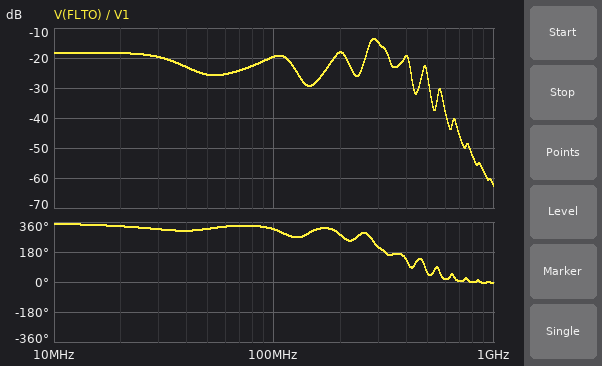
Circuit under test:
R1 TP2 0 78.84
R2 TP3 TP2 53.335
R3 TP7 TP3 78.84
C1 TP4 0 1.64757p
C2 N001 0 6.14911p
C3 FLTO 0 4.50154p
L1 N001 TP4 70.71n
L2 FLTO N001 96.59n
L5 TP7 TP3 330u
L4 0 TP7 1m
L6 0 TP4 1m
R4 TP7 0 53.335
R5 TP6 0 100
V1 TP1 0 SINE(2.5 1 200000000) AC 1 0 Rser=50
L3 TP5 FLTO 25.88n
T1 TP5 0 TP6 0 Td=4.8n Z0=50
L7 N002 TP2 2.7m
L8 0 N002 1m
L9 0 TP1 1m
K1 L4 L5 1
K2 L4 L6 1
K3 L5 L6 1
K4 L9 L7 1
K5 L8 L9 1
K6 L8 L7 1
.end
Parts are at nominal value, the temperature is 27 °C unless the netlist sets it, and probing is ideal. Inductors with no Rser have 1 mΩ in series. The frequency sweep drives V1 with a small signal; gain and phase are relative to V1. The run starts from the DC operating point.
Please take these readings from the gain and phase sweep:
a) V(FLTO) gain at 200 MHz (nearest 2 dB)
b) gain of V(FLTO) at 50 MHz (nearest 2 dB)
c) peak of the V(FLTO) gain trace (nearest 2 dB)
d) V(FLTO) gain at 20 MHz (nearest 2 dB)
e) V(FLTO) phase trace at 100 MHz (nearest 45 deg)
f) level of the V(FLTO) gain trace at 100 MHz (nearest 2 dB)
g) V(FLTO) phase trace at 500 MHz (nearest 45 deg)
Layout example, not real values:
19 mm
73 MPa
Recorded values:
-18 dB
-26 dB
-14 dB
-18 dB
315 deg
-20 dB
45 deg
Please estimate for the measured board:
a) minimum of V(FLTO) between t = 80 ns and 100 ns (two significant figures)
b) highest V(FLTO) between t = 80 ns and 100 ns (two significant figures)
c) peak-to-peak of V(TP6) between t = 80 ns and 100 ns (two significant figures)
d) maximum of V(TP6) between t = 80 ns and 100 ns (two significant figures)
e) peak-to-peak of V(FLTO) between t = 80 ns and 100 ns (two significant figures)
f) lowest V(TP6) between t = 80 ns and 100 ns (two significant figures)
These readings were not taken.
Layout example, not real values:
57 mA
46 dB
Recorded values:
-120 mV
120 mV
220 mV
110 mV
250 mV
-110 mV
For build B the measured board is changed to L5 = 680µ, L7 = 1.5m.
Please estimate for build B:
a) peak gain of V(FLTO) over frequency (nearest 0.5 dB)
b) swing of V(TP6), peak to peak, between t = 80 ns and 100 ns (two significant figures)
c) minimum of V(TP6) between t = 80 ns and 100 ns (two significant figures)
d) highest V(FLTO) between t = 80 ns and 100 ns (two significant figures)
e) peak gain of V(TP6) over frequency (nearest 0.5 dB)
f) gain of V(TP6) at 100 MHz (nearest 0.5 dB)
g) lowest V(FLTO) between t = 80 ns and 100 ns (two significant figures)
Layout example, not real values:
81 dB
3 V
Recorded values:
-12.5 dB
230 mV
-120 mV
130 mV
-15.0 dB
-19.5 dB
-130 mV
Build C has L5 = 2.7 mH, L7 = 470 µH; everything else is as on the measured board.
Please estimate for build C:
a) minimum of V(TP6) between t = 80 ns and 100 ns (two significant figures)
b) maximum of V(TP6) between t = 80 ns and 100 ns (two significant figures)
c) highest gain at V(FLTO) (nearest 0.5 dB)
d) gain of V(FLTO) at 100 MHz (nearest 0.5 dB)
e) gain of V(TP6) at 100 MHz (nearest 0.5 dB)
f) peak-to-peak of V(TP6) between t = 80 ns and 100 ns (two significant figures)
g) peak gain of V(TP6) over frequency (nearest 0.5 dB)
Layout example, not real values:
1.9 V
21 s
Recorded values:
-100 mV
100 mV
-12.0 dB
-20.0 dB
-20.5 dB
210 mV
-14.5 dB
